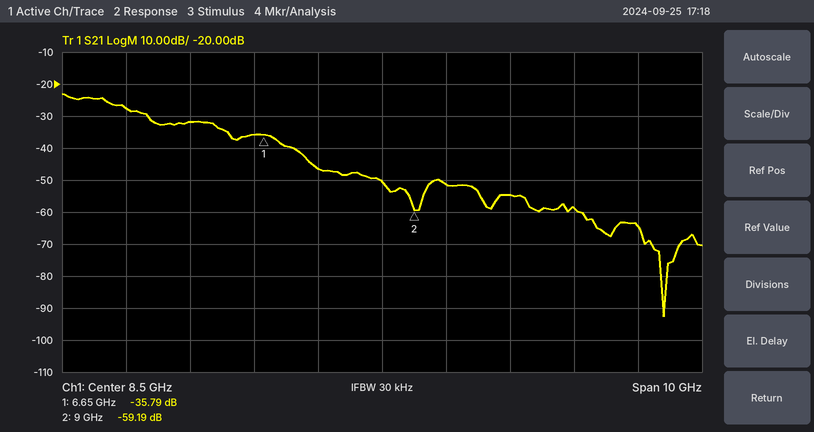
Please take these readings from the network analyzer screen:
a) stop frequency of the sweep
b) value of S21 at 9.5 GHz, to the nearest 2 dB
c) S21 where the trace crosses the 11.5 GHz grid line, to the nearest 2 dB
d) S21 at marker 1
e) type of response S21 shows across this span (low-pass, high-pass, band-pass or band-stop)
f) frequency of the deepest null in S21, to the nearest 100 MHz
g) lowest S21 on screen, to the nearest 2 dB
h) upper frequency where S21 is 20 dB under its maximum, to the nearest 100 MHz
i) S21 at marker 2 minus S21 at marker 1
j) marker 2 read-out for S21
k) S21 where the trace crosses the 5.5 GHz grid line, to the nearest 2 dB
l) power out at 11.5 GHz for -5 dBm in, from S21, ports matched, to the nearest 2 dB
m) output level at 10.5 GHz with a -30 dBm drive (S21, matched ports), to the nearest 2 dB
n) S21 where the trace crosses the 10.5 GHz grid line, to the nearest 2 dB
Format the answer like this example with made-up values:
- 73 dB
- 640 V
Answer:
- 13.5 GHz
- -52 dB
- -58 dB
- -35.79 dB
- low-pass
- 12.9 GHz
- -92 dB
- 7.3 GHz
- -23.40 dB
- -59.19 dB
- -32 dB
- -64 dBm
- -84 dBm
- -54 dB
